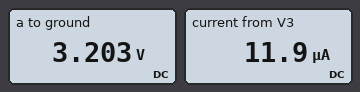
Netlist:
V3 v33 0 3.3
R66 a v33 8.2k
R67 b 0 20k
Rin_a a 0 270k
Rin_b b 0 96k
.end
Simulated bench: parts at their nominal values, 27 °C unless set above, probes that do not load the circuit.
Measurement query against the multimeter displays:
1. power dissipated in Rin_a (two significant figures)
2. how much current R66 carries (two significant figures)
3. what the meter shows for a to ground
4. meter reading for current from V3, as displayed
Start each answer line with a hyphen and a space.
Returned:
- 38 µW
- 12 µA
- 3.203 V
- 11.9 µA
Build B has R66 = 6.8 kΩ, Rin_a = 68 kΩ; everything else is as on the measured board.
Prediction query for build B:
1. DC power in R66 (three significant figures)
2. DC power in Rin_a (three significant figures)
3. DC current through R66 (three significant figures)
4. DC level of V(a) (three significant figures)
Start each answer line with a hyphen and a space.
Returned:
- 13.2 µW
- 132 µW
- 44.1 µA
- 3.00 V
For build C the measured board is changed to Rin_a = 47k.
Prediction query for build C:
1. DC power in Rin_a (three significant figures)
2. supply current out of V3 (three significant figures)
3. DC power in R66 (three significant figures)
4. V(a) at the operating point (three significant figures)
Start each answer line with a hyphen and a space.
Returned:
- 168 µW
- 59.8 µA
- 29.3 µW
- 2.81 V
